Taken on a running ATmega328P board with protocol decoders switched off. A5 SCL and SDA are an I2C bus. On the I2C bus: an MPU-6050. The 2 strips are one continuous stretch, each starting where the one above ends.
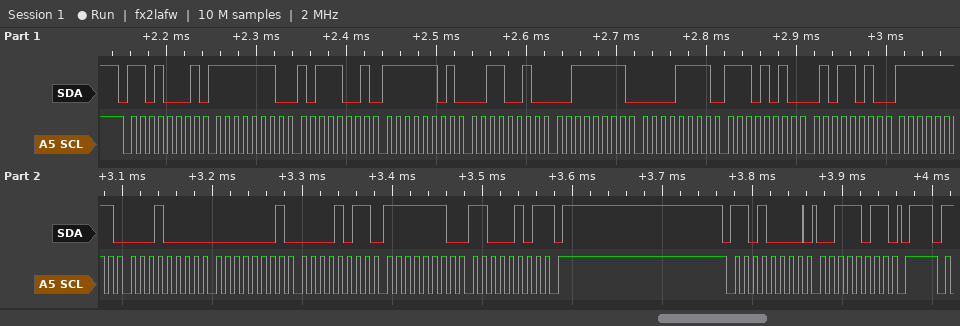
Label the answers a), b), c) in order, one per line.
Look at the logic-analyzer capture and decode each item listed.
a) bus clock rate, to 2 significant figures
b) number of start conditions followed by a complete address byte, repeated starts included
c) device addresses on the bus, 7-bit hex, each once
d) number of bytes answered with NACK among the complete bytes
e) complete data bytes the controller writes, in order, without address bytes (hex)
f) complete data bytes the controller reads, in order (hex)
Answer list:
a) 100 kHz
b) 2
c) 0x68
d) 1
e) 3B
f) FE B9 FD 32 3F 0F EA 5A FF 10 01 0B FE C5
